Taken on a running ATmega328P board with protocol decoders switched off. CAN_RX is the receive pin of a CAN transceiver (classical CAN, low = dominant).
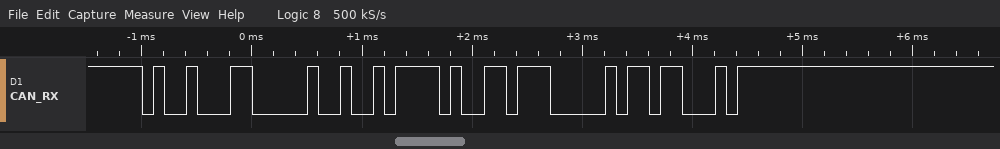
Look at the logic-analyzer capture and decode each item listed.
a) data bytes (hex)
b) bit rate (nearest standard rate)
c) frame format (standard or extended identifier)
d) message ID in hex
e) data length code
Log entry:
5E 9B
10 kbit/s
standard
0x48C
2
